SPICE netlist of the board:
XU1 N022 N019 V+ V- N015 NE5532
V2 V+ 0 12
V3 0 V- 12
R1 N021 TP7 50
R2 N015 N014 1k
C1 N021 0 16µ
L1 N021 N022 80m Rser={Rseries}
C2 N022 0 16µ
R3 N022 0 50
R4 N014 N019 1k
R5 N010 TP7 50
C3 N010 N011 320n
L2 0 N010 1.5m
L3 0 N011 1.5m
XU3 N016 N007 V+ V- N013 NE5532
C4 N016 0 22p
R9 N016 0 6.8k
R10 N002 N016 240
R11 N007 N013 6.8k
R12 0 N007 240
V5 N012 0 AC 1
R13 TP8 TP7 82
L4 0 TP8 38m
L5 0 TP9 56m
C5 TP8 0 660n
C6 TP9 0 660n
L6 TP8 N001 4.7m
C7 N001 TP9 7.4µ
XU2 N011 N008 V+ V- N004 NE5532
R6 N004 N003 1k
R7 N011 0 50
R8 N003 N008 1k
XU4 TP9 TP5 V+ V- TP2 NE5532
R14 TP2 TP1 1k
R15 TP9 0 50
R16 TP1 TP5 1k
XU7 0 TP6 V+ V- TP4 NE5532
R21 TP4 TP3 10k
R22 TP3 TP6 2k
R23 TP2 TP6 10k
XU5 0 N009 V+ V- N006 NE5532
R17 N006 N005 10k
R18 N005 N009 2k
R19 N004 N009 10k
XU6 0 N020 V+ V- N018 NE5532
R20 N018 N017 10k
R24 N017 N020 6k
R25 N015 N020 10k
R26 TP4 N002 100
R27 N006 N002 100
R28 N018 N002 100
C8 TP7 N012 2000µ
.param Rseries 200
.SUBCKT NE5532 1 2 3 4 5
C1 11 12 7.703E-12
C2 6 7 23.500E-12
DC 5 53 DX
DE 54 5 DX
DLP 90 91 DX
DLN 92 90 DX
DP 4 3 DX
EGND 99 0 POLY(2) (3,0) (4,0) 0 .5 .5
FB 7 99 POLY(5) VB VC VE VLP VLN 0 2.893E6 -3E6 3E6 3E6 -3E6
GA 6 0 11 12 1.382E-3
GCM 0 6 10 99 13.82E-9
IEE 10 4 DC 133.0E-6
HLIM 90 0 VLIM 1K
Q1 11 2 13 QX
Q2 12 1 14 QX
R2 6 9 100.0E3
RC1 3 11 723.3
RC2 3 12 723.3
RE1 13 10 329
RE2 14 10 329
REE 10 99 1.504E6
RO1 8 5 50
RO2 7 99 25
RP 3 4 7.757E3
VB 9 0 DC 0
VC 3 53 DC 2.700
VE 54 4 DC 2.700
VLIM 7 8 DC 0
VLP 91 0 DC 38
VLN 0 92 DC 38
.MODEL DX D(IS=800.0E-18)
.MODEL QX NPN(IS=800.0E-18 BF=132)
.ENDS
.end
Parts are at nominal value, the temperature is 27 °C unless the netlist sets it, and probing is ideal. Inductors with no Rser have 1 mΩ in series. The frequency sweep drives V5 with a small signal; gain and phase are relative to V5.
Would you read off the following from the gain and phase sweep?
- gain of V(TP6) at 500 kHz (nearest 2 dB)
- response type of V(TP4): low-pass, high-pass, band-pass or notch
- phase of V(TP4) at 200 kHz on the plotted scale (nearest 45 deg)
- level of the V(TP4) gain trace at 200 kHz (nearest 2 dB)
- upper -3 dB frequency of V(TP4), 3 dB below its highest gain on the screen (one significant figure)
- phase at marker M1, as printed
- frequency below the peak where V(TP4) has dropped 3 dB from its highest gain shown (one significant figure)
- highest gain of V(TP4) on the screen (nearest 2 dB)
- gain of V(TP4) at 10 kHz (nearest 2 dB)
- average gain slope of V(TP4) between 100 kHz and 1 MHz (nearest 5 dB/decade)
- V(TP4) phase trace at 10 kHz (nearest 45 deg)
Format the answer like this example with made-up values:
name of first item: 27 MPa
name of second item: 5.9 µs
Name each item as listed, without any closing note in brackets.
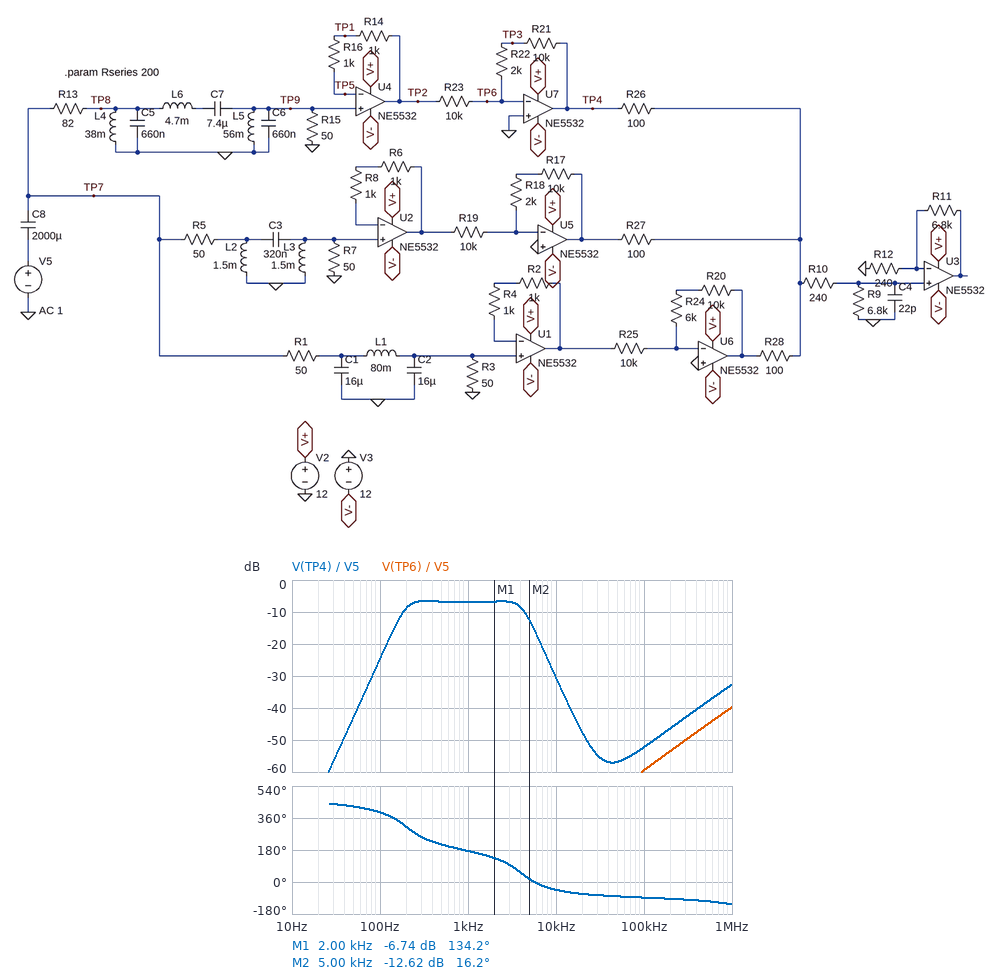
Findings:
gain of V(TP6) at 500 kHz: -46 dB
response type of V(TP4): low-pass, high-pass, band-pass or notch: band-pass
phase of V(TP4) at 200 kHz on the plotted scale: -90 deg
level of the V(TP4) gain trace at 200 kHz: -46 dB
upper -3 dB frequency of V(TP4), 3 dB below its highest gain on the screen: 4 kHz
phase at marker M1, as printed: 134.2 deg
frequency below the peak where V(TP4) has dropped 3 dB from its highest gain shown: 200 Hz
highest gain of V(TP4) on the screen: -6 dB
gain of V(TP4) at 10 kHz: -30 dB
average gain slope of V(TP4) between 100 kHz and 1 MHz: 20 dB/decade
V(TP4) phase trace at 10 kHz: -45 deg
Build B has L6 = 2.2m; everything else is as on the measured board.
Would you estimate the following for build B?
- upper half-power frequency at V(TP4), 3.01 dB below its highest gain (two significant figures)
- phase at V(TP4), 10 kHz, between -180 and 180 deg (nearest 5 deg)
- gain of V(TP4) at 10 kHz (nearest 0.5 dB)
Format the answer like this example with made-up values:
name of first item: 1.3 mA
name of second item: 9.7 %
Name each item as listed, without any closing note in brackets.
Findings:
upper half-power frequency at V(TP4), 3.01 dB below its highest gain: 6.5 kHz
phase at V(TP4), 10 kHz, between -180 and 180 deg: -40 deg
gain of V(TP4) at 10 kHz: -22.0 dB
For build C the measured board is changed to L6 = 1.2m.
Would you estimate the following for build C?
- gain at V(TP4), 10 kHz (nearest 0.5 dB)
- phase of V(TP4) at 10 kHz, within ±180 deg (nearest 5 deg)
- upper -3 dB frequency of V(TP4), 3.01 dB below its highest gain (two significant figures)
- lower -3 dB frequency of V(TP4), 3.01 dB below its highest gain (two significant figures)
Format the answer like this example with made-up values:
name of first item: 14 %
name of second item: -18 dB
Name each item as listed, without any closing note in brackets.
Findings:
gain at V(TP4), 10 kHz: -13.5 dB
phase of V(TP4) at 10 kHz, within ±180 deg: -20 deg
upper -3 dB frequency of V(TP4), 3.01 dB below its highest gain: 8.9 kHz
lower -3 dB frequency of V(TP4), 3.01 dB below its highest gain: 190 Hz
